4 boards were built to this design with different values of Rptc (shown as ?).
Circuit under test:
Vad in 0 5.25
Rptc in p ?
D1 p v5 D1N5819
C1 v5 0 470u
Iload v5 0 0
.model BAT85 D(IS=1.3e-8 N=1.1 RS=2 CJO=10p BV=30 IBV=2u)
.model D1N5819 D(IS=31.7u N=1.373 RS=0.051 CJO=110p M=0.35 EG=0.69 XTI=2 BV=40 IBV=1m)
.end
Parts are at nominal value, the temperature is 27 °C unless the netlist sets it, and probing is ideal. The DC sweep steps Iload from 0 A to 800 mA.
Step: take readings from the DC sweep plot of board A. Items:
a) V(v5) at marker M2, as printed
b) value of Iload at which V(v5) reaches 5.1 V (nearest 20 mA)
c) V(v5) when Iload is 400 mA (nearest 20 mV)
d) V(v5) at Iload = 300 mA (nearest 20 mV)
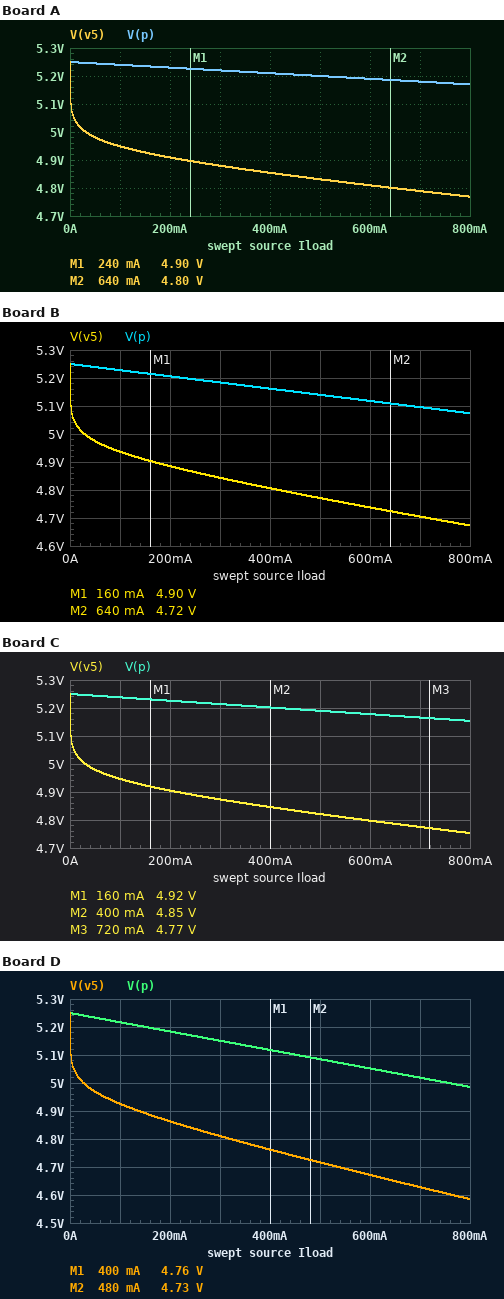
4.80 V
0 A
4.86 V
4.88 V
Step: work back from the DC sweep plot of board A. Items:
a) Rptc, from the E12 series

0.1 Ω
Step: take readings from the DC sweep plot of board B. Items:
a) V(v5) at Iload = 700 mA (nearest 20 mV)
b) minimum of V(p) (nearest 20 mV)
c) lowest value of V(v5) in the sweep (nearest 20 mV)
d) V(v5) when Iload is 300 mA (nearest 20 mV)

4.70 V
5.08 V
4.68 V
4.84 V
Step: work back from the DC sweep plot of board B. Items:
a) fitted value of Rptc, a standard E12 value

0.22 Ω
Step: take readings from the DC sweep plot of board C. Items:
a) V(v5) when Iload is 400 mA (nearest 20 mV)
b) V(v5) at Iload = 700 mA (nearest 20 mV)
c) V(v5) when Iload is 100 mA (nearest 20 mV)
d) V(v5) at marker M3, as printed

4.84 V
4.78 V
4.94 V
4.77 V
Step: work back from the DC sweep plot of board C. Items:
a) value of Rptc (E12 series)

0.12 Ω
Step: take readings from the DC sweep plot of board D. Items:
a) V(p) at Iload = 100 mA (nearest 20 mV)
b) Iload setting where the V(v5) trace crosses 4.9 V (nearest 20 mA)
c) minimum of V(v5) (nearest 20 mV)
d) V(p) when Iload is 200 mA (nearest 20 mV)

5.22 V
140 mA
4.58 V
5.18 V
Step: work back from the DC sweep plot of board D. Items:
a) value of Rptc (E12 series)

0.33 Ω
